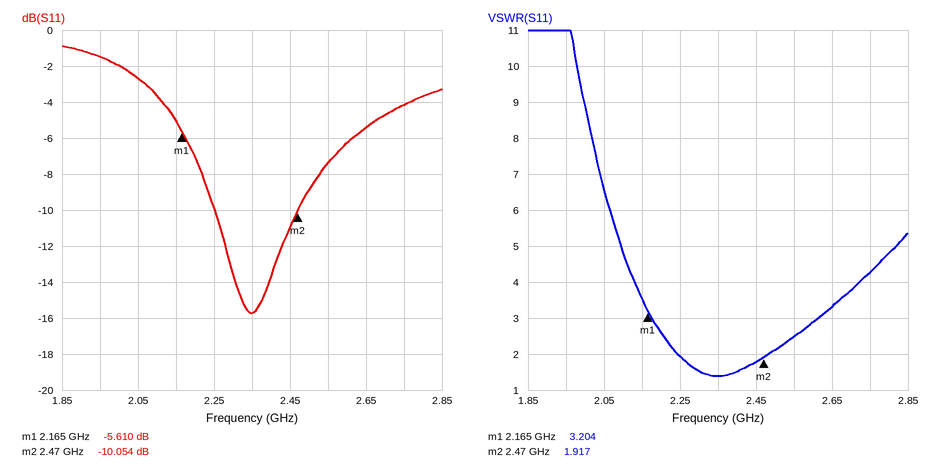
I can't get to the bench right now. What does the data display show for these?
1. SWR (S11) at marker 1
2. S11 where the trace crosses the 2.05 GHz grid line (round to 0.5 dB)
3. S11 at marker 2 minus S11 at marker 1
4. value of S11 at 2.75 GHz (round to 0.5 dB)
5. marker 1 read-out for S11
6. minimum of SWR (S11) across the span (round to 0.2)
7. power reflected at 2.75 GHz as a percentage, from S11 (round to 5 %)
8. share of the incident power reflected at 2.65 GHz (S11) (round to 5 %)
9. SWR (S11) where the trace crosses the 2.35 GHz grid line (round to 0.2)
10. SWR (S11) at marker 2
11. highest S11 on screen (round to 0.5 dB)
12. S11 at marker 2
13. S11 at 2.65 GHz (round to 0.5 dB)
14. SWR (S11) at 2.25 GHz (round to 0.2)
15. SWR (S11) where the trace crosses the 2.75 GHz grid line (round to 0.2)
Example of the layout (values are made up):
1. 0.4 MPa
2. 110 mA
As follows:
1. 3.204
2. -2.5 dB
3. -4.444 dB
4. -4.0 dB
5. -5.610 dB
6. 1.4
7. 40 %
8. 30 %
9. 1.4
10. 1.917
11. -1.0 dB
12. -10.054 dB
13. -5.5 dB
14. 2.0
15. 4.2
